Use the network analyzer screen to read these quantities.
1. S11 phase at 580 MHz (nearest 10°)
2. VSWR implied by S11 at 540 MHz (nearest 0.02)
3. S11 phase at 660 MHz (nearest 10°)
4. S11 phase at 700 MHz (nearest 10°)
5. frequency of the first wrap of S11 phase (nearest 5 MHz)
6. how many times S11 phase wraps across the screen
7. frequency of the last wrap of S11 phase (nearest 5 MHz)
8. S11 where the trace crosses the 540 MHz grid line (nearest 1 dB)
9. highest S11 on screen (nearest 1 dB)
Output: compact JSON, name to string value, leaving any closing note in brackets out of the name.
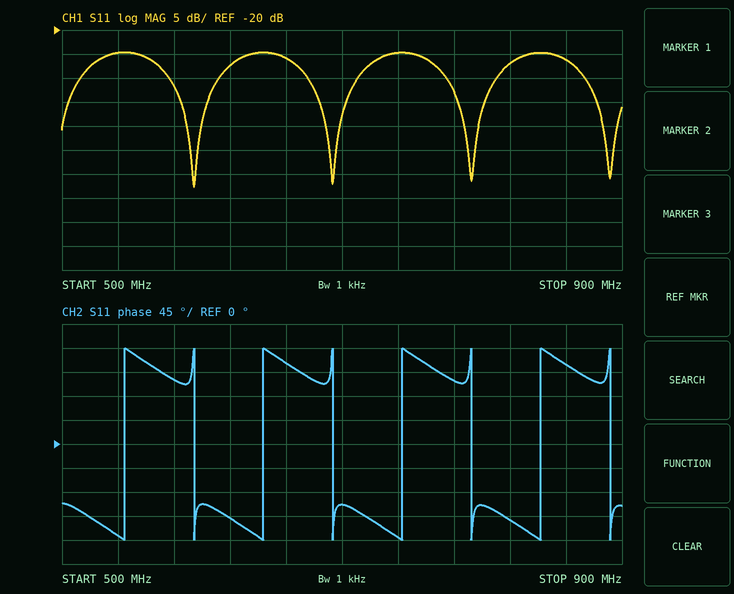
{"S11 phase at 580 MHz": "120°", "VSWR implied by S11 at 540 MHz": "1.12", "S11 phase at 660 MHz": "150°", "S11 phase at 700 MHz": "-110°", "frequency of the first wrap of S11 phase": "545 MHz", "how many times S11 phase wraps across the screen": "8", "frequency of the last wrap of S11 phase": "890 MHz", "S11 where the trace crosses the 540 MHz grid line": "-25 dB", "highest S11 on screen": "-25 dB"}
